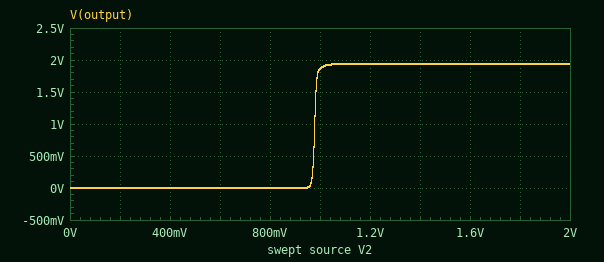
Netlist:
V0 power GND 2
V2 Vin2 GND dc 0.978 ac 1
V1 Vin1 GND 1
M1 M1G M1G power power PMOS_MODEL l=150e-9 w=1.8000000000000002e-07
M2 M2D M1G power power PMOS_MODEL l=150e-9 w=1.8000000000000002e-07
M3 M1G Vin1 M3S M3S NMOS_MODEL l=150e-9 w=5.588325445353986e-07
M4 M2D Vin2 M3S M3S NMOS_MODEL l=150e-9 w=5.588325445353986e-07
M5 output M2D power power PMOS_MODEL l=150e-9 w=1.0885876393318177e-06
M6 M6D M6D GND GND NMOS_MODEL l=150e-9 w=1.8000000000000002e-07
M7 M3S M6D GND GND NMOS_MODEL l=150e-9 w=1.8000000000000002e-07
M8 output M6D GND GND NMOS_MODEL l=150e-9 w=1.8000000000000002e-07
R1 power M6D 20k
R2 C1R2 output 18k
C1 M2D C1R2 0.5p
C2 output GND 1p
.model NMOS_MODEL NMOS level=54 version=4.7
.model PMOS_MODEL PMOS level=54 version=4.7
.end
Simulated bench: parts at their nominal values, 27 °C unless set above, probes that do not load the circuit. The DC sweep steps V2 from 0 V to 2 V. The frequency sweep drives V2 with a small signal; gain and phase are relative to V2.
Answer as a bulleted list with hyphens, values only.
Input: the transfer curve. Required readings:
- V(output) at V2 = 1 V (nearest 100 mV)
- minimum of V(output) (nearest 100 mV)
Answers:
- 1.9 V
- 0 V
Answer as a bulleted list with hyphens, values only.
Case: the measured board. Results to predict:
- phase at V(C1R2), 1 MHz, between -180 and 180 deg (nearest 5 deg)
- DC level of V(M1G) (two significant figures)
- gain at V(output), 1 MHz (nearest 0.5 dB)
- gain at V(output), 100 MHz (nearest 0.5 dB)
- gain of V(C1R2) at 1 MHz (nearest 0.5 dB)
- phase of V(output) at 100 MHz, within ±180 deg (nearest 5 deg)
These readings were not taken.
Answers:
- -70 deg
- 1.1 V
- 34.0 dB
- 2.0 dB
- 34.0 dB
- -75 deg
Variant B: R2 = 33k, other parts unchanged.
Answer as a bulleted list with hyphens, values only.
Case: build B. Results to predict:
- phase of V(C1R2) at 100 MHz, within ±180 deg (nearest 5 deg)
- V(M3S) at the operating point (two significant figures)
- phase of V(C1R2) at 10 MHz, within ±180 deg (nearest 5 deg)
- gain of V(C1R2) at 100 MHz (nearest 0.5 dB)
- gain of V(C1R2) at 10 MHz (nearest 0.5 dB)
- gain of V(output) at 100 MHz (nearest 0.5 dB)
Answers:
- -165 deg
- 500 mV
- -110 deg
- 13.0 dB
- 16.0 dB
- 6.5 dB
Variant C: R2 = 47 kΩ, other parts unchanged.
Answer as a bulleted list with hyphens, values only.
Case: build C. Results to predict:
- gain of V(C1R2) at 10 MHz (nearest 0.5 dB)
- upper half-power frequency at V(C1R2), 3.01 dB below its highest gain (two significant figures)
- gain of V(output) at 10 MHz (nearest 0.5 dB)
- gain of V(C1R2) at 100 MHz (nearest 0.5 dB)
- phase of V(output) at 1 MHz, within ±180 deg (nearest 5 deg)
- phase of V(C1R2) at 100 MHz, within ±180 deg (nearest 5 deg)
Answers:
- 16.5 dB
- 430 kHz
- 19.0 dB
- 14.5 dB
- -60 deg
- -170 deg
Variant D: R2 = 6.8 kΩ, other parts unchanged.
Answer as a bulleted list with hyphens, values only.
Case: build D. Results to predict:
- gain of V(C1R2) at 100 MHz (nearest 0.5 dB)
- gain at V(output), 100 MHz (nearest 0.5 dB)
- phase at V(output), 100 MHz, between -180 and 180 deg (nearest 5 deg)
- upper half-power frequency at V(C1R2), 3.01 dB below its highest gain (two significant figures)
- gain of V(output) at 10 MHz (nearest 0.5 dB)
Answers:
- 3.5 dB
- -6.5 dB
- -100 deg
- 450 kHz
- 15.0 dB
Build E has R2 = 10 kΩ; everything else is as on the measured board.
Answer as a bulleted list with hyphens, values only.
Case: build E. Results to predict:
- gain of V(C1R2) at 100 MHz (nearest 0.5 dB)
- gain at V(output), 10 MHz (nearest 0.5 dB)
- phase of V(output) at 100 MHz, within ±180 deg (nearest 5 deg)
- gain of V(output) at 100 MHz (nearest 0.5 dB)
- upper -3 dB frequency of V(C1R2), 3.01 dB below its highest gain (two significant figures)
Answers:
- 5.5 dB
- 15.0 dB
- -85 deg
- -3.0 dB
- 450 kHz
